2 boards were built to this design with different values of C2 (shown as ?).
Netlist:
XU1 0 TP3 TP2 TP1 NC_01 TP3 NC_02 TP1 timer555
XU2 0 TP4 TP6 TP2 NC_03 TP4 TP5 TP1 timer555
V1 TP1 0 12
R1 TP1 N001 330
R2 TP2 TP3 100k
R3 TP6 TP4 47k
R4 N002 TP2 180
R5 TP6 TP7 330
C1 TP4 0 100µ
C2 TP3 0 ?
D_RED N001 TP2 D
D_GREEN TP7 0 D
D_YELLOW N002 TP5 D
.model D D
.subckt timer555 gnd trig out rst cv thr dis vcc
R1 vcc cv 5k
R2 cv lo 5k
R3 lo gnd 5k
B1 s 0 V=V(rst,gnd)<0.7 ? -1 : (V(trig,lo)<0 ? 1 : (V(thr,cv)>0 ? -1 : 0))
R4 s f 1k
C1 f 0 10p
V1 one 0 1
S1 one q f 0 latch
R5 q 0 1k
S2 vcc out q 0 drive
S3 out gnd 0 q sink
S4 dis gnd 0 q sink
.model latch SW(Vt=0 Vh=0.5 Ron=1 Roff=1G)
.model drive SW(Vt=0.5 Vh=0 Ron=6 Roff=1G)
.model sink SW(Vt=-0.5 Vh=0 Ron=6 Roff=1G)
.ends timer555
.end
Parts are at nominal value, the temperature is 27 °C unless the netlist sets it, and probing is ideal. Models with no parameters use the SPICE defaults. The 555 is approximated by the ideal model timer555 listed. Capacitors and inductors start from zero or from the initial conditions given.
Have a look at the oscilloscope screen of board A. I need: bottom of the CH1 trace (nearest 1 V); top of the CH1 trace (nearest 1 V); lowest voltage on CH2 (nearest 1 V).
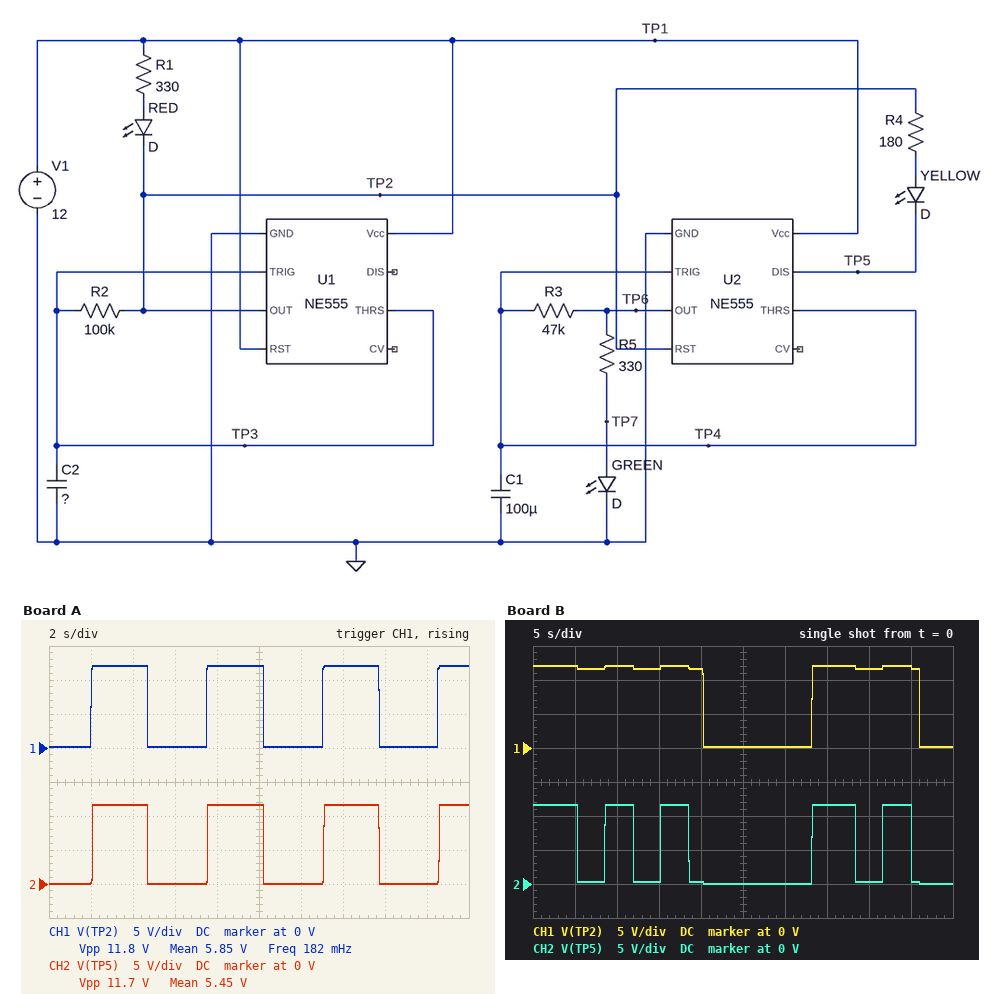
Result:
0 V
12 V
0 V
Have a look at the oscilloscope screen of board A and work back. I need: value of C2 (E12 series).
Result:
39 µF
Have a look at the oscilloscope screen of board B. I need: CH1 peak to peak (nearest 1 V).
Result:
12 V
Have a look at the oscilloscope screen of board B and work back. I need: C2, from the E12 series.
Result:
180 µF
